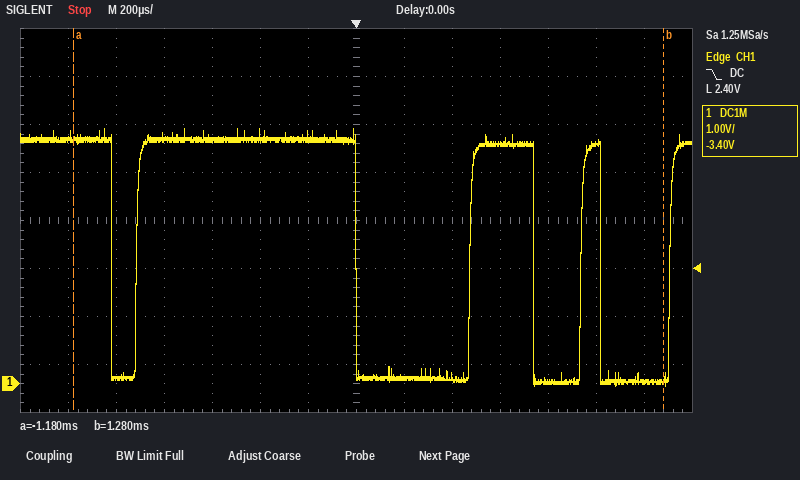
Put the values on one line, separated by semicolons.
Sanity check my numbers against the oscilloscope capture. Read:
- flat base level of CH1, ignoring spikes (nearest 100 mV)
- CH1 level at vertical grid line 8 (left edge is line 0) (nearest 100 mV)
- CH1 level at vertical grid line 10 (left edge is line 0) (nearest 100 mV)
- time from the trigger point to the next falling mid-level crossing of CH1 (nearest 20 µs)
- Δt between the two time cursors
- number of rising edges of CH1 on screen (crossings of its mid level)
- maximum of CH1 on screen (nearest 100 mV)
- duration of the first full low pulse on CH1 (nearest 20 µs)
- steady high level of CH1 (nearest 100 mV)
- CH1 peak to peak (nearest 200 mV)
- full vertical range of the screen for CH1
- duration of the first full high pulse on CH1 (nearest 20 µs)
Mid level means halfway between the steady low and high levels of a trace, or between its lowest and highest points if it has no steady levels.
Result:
100 mV; 100 mV; 5.0 V; 740 µs; 2.46 ms; 4; 5.3 V; 100 µs; 5.1 V; 5.4 V; 8 V; 920 µs
